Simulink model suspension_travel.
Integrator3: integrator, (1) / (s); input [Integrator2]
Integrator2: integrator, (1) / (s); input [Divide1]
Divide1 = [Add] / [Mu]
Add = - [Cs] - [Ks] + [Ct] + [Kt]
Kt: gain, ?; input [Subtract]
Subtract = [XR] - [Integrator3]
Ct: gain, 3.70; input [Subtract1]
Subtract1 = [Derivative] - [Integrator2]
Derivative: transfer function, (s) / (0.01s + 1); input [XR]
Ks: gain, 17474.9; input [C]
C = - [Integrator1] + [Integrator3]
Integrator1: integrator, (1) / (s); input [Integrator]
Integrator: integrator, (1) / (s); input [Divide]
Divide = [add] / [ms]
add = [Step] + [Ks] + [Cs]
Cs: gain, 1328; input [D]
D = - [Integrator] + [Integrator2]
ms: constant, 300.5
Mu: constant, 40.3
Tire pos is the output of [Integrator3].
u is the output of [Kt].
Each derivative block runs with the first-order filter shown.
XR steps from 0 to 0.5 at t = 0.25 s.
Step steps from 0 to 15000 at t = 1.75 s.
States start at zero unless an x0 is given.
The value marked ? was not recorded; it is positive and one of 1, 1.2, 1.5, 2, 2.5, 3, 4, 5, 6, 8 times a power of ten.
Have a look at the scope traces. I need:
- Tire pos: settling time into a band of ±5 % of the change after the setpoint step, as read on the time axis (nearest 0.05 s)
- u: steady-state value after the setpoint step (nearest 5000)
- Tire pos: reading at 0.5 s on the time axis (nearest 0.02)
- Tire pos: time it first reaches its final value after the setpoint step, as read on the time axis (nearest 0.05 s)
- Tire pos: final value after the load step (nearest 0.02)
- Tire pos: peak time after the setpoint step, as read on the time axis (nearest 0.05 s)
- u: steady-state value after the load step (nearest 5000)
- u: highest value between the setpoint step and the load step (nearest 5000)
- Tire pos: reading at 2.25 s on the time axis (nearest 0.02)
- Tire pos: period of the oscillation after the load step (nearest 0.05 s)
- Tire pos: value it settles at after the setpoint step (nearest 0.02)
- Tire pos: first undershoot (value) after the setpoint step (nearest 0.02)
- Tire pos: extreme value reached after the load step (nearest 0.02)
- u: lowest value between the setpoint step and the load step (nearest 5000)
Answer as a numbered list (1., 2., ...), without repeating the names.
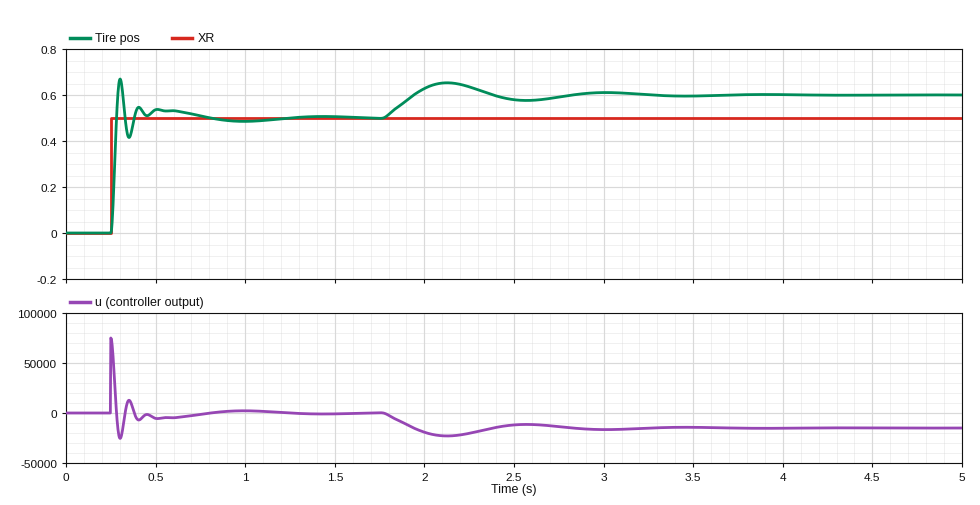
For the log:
1. 0.65 s
2. 0
3. 0.54
4. 0.30 s
5. 0.60
6. 0.30 s
7. -15000
8. 75000
9. 0.64
10. 0.90 s
11. 0.50
12. 0.42
13. 0.66
14. -25000
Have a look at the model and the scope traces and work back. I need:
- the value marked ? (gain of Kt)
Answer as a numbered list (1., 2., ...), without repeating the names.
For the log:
1. 150000
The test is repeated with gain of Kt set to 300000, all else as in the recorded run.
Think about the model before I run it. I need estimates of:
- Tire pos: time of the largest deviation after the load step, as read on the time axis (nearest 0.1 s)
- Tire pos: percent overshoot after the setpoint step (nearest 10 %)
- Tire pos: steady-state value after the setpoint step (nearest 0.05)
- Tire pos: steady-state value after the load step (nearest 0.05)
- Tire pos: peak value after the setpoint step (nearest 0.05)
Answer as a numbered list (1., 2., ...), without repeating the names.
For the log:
1. 2.1 s
2. 50 %
3. 0.50
4. 0.55
5. 0.75
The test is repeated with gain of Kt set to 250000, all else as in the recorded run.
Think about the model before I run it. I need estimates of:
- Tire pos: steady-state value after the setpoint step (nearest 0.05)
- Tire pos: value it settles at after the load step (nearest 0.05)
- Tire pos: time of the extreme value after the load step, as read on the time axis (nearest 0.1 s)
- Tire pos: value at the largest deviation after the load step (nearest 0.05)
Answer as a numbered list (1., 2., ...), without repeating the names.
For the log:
1. 0.50
2. 0.55
3. 2.1 s
4. 0.60
